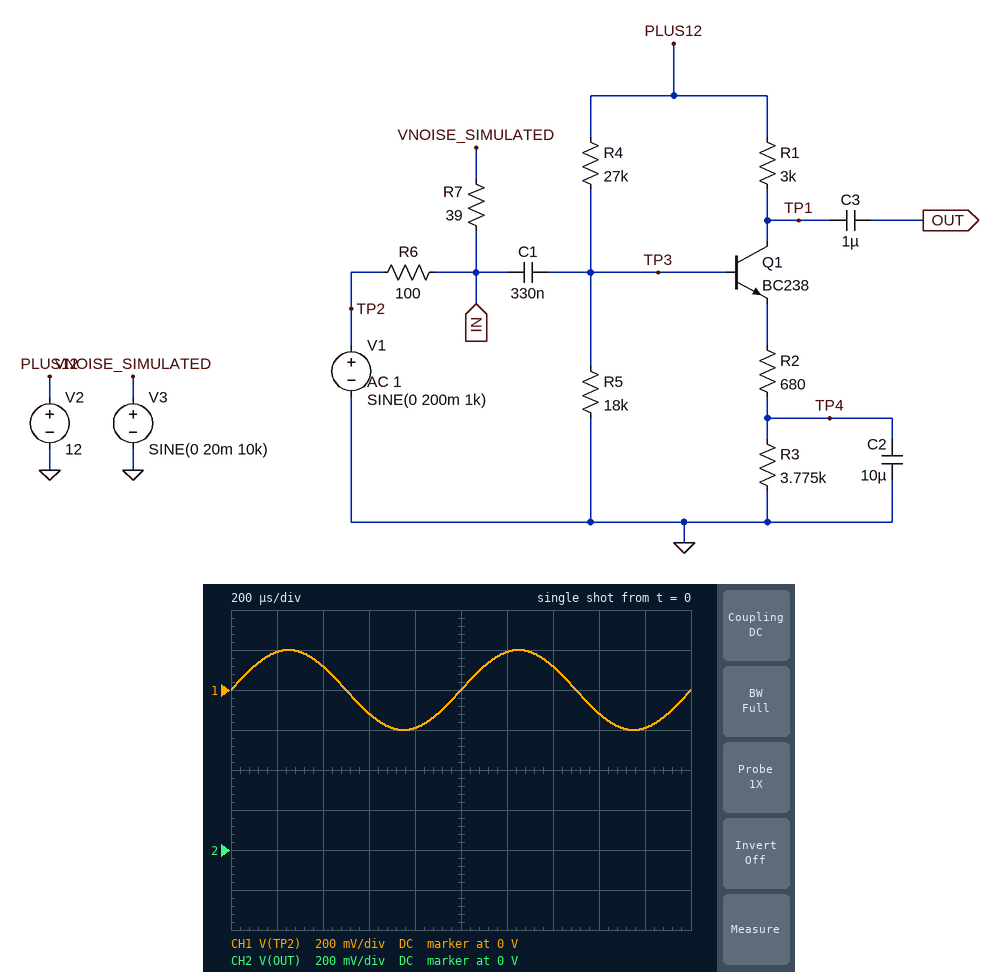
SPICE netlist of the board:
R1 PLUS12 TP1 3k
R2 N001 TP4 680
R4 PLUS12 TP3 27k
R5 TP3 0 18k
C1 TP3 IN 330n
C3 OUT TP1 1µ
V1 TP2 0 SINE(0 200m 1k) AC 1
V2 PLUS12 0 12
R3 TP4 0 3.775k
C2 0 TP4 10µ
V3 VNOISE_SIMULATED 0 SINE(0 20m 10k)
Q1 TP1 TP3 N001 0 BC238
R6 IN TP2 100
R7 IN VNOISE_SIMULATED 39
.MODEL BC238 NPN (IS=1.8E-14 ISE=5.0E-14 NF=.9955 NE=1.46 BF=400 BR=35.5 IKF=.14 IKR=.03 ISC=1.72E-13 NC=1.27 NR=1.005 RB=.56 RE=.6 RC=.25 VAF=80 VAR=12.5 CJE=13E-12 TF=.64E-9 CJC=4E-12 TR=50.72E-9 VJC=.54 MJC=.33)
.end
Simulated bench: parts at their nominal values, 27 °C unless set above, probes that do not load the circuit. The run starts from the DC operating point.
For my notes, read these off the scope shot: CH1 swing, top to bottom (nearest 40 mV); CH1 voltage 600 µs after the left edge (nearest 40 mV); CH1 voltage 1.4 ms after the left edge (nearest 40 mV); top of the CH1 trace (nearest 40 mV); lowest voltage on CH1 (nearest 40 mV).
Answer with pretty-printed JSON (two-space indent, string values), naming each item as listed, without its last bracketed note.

{
  "CH1 swing, top to bottom": "400 mV",
  "CH1 voltage 600 µs after the left edge": "-120 mV",
  "CH1 voltage 1.4 ms after the left edge": "120 mV",
  "top of the CH1 trace": "200 mV",
  "lowest voltage on CH1": "-200 mV"
}
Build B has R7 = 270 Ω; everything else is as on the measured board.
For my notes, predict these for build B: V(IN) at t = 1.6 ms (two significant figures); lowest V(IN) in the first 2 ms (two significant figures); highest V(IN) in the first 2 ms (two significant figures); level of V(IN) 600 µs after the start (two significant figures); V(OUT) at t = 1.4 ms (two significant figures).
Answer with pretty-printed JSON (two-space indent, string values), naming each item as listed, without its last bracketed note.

{
  "V(IN) at t = 1.6 ms": "-65 mV",
  "lowest V(IN) in the first 2 ms": "-130 mV",
  "highest V(IN) in the first 2 ms": "180 mV",
  "level of V(IN) 600 µs after the start": "-58 mV",
  "V(OUT) at t = 1.4 ms": "7.9 V"
}
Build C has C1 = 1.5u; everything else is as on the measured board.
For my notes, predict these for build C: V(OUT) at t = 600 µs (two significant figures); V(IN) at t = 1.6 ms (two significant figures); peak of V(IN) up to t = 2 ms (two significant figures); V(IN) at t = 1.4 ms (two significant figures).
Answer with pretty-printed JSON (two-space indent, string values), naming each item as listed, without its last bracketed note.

{
  "V(OUT) at t = 600 µs": "12 V",
  "V(IN) at t = 1.6 ms": "-22 mV",
  "peak of V(IN) up to t = 2 ms": "82 mV",
  "V(IN) at t = 1.4 ms": "44 mV"
}
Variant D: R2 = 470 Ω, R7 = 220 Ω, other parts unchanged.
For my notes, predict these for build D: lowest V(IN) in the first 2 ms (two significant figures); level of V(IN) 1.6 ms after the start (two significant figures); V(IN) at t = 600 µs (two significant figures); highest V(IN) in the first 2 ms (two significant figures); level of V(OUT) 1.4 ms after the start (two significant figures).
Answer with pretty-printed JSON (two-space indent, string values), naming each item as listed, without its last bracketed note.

{
  "lowest V(IN) in the first 2 ms": "-120 mV",
  "level of V(IN) 1.6 ms after the start": "-61 mV",
  "V(IN) at t = 600 µs": "-55 mV",
  "highest V(IN) in the first 2 ms": "170 mV",
  "level of V(OUT) 1.4 ms after the start": "6.3 V"
}
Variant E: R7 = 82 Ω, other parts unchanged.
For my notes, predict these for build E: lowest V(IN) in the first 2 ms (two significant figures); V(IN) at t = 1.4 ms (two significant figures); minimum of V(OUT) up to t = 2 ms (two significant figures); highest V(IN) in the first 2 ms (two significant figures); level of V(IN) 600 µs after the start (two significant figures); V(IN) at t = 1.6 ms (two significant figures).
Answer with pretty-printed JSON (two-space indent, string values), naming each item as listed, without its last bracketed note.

{
  "lowest V(IN) in the first 2 ms": "-88 mV",
  "V(IN) at t = 1.4 ms": "66 mV",
  "minimum of V(OUT) up to t = 2 ms": "6.5 V",
  "highest V(IN) in the first 2 ms": "120 mV",
  "level of V(IN) 600 µs after the start": "-36 mV",
  "V(IN) at t = 1.6 ms": "-40 mV"
}
